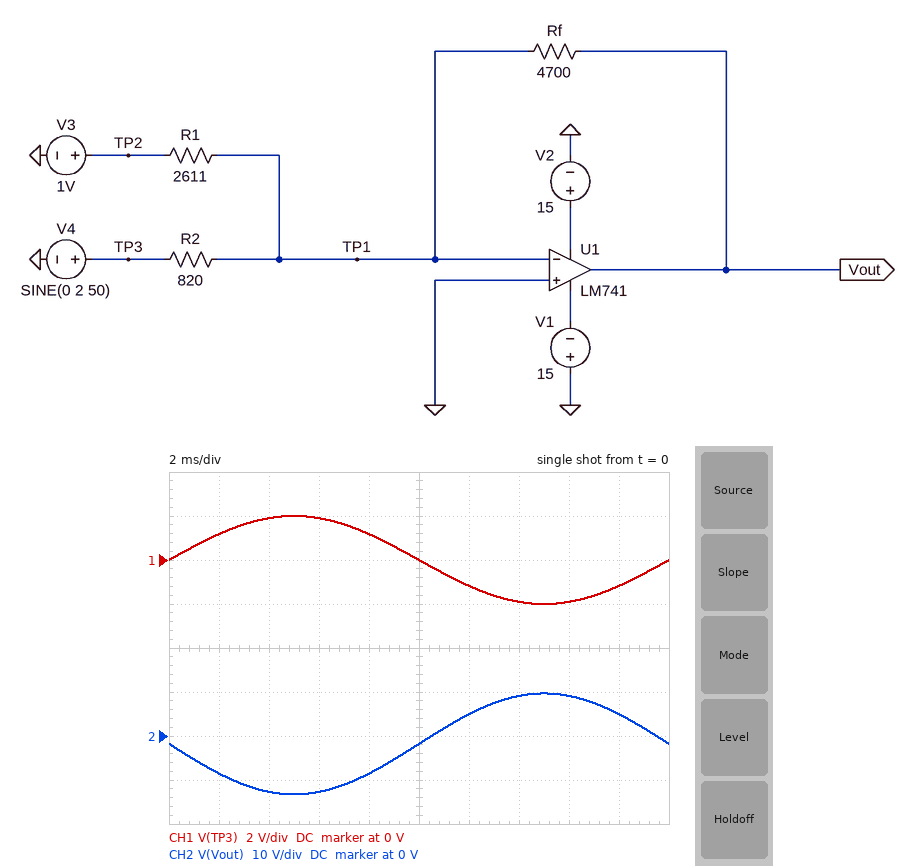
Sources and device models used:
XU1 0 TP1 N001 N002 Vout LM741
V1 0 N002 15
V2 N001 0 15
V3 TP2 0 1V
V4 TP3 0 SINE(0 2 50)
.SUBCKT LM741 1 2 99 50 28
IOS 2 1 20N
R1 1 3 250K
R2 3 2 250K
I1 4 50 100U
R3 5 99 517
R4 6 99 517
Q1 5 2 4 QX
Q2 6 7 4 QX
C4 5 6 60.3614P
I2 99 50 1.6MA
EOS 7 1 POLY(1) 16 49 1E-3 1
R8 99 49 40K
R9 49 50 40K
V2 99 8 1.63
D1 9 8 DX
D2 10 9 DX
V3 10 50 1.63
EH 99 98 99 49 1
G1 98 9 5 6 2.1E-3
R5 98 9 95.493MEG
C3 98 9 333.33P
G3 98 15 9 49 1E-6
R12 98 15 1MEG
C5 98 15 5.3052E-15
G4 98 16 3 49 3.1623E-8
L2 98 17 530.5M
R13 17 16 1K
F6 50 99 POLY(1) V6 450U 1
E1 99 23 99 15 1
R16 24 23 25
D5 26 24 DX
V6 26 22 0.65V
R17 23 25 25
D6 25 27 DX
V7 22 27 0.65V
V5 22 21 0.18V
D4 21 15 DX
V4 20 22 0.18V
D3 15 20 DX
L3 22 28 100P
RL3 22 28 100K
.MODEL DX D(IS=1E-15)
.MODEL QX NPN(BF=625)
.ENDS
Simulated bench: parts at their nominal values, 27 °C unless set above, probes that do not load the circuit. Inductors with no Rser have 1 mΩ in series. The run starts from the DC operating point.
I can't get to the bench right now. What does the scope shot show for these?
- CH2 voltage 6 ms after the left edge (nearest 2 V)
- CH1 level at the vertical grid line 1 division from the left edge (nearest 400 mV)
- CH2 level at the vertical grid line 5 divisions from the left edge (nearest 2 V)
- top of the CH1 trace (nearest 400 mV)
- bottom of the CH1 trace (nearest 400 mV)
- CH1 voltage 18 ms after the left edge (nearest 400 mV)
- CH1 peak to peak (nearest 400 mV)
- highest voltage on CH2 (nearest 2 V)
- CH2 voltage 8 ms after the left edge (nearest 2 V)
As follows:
-12 V
1.2 V
-2 V
2.0 V
-2.0 V
-1.2 V
4.0 V
10 V
-8 V
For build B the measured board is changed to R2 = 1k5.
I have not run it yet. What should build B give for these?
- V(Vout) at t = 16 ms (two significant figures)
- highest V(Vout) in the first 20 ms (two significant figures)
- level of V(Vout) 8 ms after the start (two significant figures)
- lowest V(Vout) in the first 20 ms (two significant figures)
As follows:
4.2 V
4.5 V
-5.5 V
-8.1 V
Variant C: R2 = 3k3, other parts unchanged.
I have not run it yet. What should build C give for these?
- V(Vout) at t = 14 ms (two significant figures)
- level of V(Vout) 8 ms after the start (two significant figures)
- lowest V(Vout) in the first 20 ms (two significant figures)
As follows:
910 mV
-3.5 V
-4.6 V
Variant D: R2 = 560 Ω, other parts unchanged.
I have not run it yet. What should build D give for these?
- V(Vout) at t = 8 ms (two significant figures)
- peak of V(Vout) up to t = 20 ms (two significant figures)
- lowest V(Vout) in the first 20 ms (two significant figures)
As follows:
-12 V
14 V
-14 V
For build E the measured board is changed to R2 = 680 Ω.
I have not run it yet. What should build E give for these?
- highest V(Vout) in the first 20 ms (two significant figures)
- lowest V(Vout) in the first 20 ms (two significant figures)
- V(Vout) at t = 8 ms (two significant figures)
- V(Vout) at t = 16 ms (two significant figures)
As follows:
12 V
-14 V
-9.9 V
11 V
